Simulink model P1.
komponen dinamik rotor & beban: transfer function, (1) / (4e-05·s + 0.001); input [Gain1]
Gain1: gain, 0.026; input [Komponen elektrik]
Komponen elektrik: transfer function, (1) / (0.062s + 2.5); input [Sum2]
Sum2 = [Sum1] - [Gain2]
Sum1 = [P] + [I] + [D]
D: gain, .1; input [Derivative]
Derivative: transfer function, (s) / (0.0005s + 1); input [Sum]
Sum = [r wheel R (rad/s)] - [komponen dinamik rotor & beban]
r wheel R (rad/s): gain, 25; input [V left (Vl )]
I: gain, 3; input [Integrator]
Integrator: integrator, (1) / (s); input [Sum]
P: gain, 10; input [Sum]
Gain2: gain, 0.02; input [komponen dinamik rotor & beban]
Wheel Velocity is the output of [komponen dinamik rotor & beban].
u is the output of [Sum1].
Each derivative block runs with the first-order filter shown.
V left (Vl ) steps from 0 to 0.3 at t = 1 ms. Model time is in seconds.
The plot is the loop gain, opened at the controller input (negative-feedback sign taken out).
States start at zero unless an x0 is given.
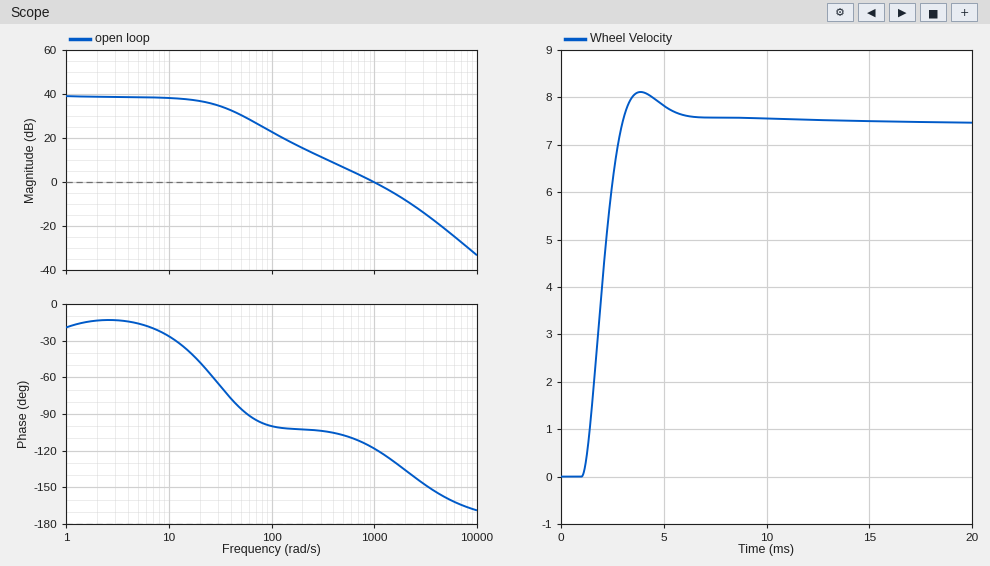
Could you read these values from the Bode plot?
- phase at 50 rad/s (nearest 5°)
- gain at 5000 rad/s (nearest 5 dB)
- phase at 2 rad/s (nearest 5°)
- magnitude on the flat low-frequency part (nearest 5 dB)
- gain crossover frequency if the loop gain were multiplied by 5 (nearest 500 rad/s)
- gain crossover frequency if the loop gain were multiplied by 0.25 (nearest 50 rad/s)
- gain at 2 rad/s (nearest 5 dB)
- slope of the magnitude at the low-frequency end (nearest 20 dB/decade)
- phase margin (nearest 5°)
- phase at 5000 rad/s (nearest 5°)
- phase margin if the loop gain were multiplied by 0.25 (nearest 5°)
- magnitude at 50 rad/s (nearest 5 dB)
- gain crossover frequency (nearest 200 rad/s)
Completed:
-85°
-20 dB
-15°
40 dB
3000 rad/s
300 rad/s
40 dB
0 dB/decade
60°
-160°
75°
30 dB
1000 rad/s
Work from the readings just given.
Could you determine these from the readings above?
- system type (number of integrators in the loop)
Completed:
0
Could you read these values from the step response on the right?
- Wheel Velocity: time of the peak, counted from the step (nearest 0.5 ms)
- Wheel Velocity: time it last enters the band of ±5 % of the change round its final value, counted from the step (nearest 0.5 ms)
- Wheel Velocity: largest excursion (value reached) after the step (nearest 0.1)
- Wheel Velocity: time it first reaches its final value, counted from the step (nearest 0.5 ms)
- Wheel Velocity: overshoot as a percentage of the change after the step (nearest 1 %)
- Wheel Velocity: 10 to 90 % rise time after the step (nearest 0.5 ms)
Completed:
3.0 ms
4.0 ms
8.1
2.0 ms
9 %
1.5 ms
